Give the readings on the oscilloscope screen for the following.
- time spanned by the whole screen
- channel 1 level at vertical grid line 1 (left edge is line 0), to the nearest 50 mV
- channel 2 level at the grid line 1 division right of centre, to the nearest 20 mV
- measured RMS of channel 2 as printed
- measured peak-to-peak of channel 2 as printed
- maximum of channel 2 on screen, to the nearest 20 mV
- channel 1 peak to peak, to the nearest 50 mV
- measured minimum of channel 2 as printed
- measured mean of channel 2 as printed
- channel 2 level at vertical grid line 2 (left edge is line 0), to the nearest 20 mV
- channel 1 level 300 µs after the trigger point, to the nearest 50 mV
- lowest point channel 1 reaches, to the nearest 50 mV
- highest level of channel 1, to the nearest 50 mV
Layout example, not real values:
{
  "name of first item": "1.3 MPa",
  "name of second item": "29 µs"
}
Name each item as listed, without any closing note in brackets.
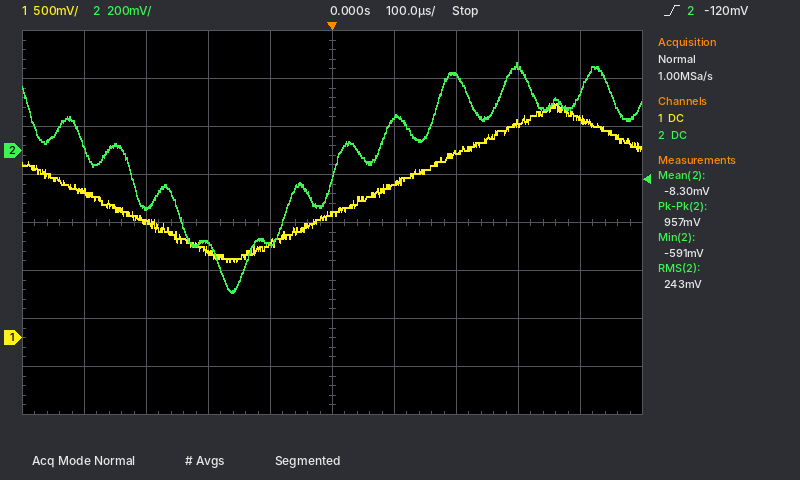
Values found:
{
  "time spanned by the whole screen": "1 ms",
  "channel 1 level at vertical grid line 1 (left edge is line 0), to the nearest 50 mV": "1.50 V",
  "channel 2 level at the grid line 1 division right of centre, to the nearest 20 mV": "140 mV",
  "measured RMS of channel 2 as printed": "243 mV",
  "measured peak-to-peak of channel 2 as printed": "957 mV",
  "maximum of channel 2 on screen, to the nearest 20 mV": "360 mV",
  "channel 1 peak to peak, to the nearest 50 mV": "1.65 V",
  "measured minimum of channel 2 as printed": "-591 mV",
  "measured mean of channel 2 as printed": "-8.30 mV",
  "channel 2 level at vertical grid line 2 (left edge is line 0), to the nearest 20 mV": "-240 mV",
  "channel 1 level 300 µs after the trigger point, to the nearest 50 mV": "2.25 V",
  "lowest point channel 1 reaches, to the nearest 50 mV": "800 mV",
  "highest level of channel 1, to the nearest 50 mV": "2.45 V"
}
